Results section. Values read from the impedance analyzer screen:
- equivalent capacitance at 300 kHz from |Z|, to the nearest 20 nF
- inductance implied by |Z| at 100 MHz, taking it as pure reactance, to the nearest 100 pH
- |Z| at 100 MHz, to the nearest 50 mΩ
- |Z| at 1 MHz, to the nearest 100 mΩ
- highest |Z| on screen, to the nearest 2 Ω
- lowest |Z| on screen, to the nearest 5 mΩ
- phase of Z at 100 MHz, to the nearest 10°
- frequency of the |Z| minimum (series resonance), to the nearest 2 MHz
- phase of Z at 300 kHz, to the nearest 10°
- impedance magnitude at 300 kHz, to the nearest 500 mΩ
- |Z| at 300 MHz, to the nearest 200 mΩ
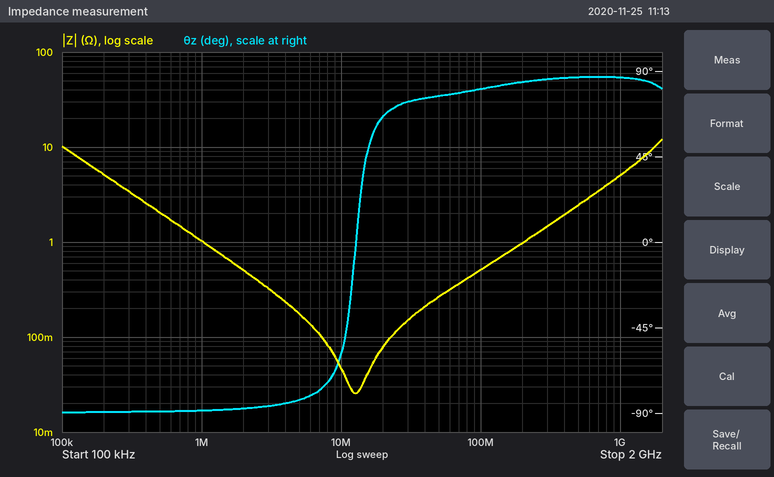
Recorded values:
160 nF
800 pH
500 mΩ
1.0 Ω
12 Ω
25 mΩ
80°
12 MHz
-90°
3.5 Ω
1.4 Ω
